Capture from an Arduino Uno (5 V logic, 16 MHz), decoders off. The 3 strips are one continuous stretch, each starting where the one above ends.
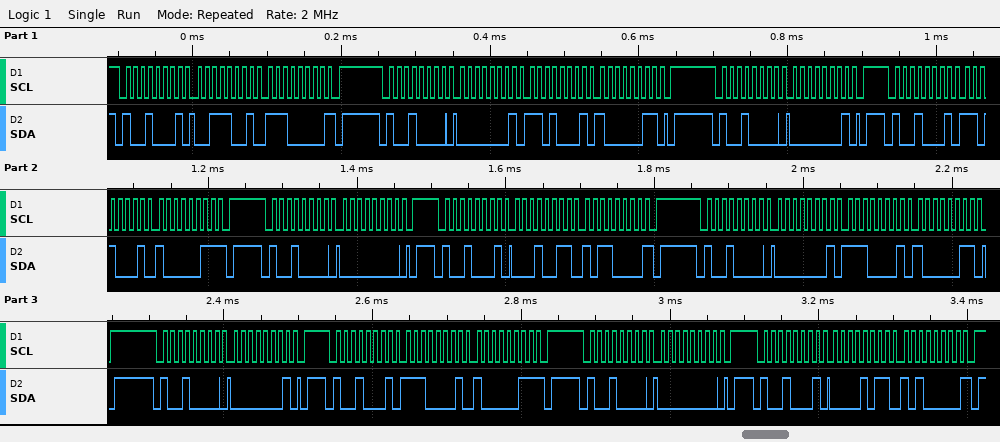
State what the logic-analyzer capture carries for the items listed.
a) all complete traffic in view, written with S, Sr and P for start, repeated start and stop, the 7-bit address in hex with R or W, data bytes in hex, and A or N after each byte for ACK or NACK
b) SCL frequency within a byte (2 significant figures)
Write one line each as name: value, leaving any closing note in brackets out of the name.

all complete traffic in view, written with S, Sr and P for start, repeated start and stop, the 7-bit address in hex with R or W, data bytes in hex, and A or N after each byte for ACK or NACK: S 48R A 39 A E0 N P S 48W A 01 A D1 A 83 A P S 48W A 01 A P S 48R A D1 A 83 N P S 48W A 00 A P S 48R A 13 A B0 N P S 48W A 01 A E1 A 83 A P S 48W A 01 A P S 48R A E1 A 83 N P S 48W A 00 A P S 48R A 0B A A0 N P
SCL frequency within a byte: 100 kHz
